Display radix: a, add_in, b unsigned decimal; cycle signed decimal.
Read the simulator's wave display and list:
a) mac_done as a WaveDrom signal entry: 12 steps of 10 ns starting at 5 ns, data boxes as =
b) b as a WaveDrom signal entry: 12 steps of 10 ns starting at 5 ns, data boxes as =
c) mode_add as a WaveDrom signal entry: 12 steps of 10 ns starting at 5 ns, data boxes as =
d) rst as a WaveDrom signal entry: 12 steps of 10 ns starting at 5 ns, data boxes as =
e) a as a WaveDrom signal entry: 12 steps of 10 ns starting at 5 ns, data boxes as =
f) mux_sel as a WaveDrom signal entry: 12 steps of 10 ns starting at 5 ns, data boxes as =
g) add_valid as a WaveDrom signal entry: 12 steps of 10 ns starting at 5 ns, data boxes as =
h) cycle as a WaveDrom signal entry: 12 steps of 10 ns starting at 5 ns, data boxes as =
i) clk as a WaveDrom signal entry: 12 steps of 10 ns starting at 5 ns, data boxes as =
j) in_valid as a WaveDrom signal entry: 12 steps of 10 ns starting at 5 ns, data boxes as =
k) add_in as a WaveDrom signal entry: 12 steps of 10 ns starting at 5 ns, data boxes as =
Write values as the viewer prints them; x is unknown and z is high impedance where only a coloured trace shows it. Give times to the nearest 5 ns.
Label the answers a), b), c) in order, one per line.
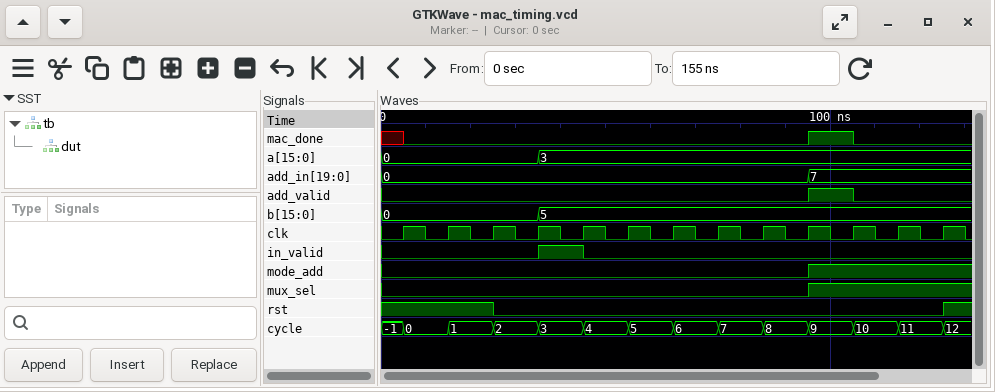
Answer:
a) {name: 'mac_done', wave: '0........10.'}
b) {name: 'b', wave: '=..=........', data: '0 5'}
c) {name: 'mode_add', wave: '0........1..'}
d) {name: 'rst', wave: '1.0.........'}
e) {name: 'a', wave: '=..=........', data: '0 3'}
f) {name: 'mux_sel', wave: '0........1..'}
g) {name: 'add_valid', wave: '0........10.'}
h) {name: 'cycle', wave: '============', data: '0 1 2 3 4 5 6 7 8 9 10 11'}
i) {name: 'clk', wave: 'p...........'}
j) {name: 'in_valid', wave: '0..10.......'}
k) {name: 'add_in', wave: '=........=..', data: '0 7'}
